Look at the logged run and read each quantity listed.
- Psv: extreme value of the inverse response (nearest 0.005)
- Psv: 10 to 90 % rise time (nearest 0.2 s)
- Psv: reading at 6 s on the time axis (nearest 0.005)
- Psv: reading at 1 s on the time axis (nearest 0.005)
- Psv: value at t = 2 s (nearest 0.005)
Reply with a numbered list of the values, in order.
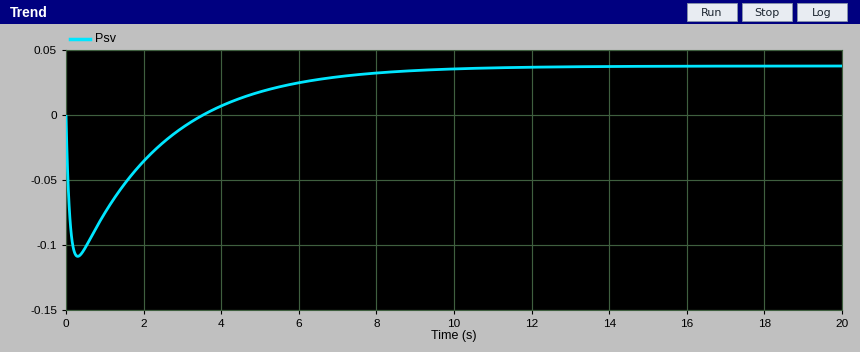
1. -0.110
2. 5.0 s
3. 0.025
4. -0.075
5. -0.035
